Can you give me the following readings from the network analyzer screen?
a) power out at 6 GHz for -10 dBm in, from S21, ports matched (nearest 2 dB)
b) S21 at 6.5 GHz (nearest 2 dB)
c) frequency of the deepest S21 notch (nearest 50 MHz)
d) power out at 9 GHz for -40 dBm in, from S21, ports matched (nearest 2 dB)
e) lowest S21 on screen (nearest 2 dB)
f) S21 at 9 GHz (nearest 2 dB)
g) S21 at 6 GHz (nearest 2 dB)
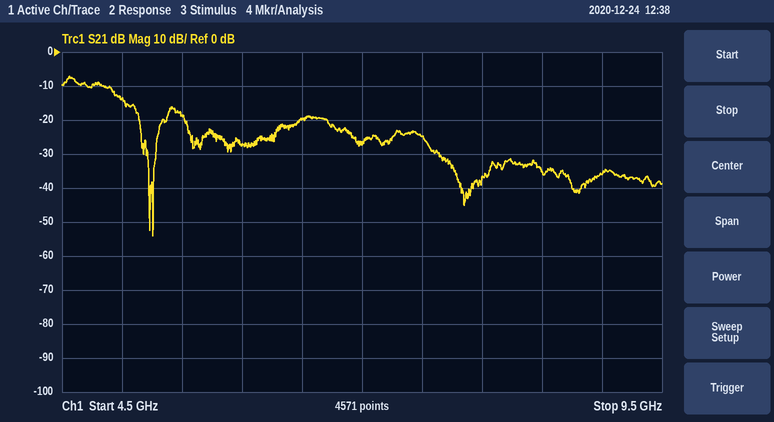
-38 dBm
-20 dB
5.25 GHz
-76 dBm
-54 dB
-36 dB
-28 dB
